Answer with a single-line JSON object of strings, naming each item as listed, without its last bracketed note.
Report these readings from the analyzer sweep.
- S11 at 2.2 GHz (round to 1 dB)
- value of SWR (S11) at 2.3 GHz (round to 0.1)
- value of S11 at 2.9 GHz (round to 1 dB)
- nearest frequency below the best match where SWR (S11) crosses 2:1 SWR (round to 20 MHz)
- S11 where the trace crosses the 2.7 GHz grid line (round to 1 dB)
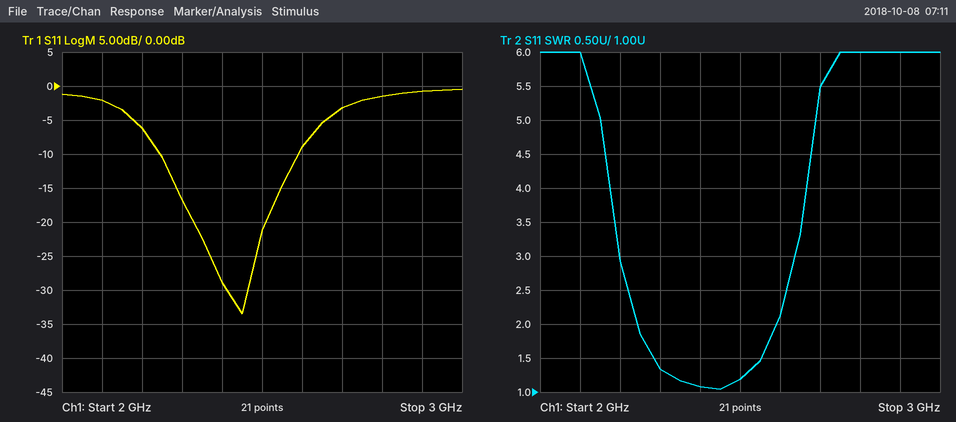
{"S11 at 2.2 GHz": "-6 dB", "value of SWR (S11) at 2.3 GHz": "1.3", "value of S11 at 2.9 GHz": "-1 dB", "nearest frequency below the best match where SWR (S11) crosses 2:1 SWR": "2.24 GHz", "S11 where the trace crosses the 2.7 GHz grid line": "-3 dB"}
